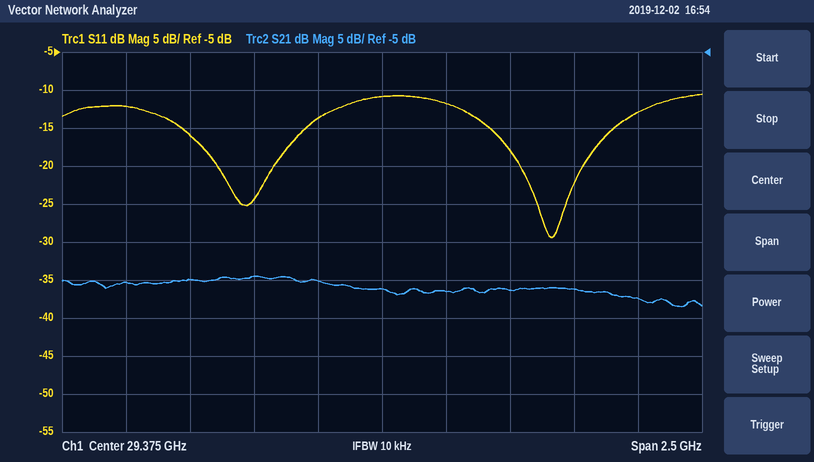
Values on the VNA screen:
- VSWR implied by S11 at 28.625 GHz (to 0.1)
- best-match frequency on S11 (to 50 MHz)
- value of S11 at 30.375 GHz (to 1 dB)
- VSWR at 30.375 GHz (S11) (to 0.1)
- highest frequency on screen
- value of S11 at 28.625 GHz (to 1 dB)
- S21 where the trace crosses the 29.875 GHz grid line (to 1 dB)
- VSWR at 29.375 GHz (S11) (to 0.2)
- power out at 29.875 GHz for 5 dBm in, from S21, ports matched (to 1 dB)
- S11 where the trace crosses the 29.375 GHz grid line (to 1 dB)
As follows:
1.4
30.05 GHz
-13 dB
1.6
30.625 GHz
-16 dB
-36 dB
1.8
-31 dBm
-11 dB
